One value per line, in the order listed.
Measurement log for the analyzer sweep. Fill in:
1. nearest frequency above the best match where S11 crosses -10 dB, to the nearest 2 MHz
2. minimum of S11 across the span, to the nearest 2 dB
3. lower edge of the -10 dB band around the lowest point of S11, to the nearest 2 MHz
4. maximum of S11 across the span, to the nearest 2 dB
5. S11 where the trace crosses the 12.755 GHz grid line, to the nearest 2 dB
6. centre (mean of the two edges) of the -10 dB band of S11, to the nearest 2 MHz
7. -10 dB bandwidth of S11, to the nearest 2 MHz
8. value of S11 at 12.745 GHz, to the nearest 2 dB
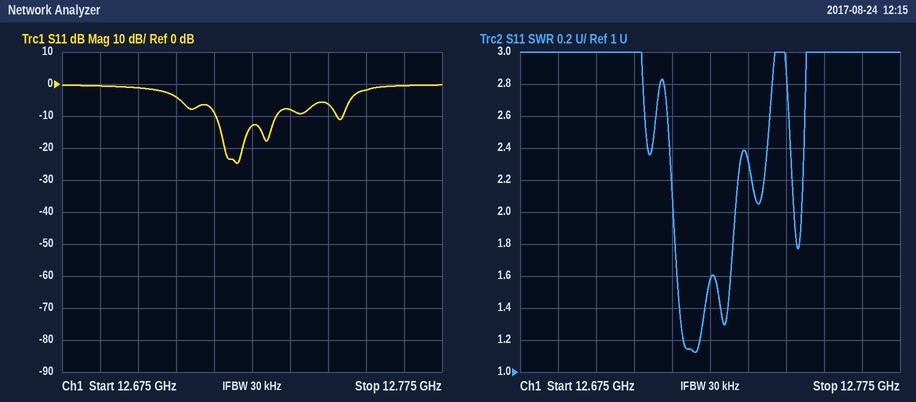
12.732 GHz
-24 dB
12.716 GHz
0 dB
-2 dB
12.724 GHz
16 MHz
-6 dB
